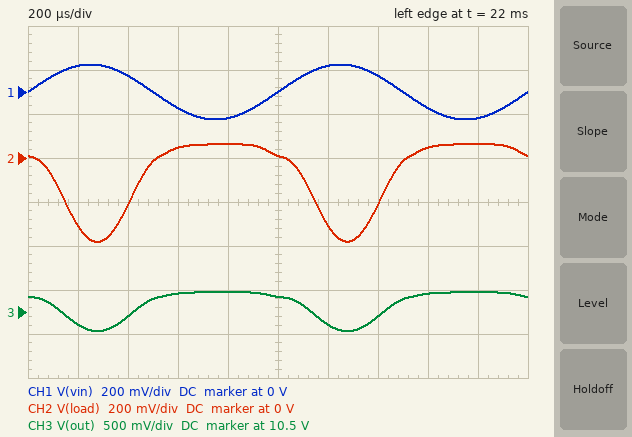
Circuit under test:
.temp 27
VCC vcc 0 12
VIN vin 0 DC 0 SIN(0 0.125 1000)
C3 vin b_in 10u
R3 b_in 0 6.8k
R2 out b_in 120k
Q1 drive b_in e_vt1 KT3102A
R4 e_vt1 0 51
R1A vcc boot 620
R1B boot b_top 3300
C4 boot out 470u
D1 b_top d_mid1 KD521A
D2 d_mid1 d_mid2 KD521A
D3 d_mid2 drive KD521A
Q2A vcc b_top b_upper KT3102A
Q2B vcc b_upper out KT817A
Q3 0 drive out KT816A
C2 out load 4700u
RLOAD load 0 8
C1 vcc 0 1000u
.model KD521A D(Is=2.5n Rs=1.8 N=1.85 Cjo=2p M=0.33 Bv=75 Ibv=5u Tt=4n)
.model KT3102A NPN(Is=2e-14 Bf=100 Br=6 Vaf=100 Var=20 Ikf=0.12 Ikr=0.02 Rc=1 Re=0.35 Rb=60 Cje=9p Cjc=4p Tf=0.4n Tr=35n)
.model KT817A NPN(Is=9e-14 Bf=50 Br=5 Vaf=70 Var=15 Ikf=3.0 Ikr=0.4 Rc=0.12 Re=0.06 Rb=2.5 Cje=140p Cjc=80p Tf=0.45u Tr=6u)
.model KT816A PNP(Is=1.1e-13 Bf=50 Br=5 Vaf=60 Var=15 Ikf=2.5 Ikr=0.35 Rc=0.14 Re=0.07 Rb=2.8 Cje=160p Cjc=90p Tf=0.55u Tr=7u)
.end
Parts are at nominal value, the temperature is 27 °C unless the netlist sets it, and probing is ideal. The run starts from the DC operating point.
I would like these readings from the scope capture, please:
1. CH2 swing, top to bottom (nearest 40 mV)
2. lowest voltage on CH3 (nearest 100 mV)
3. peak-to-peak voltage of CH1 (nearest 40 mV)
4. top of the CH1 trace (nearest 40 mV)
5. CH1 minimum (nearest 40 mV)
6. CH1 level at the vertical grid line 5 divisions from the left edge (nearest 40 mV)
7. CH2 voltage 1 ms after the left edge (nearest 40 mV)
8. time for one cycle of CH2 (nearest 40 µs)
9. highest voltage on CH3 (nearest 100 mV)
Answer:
440 mV
10.3 V
240 mV
120 mV
-120 mV
0 V
0 V
1.00 ms
10.7 V
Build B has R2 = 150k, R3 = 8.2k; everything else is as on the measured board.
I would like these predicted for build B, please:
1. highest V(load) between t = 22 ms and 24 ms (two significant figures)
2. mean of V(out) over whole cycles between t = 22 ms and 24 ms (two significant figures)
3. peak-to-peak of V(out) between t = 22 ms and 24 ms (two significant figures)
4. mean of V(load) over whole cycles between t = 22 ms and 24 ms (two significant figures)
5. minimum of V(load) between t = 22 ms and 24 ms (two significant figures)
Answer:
11 mV
11 V
340 mV
-78 mV
-330 mV
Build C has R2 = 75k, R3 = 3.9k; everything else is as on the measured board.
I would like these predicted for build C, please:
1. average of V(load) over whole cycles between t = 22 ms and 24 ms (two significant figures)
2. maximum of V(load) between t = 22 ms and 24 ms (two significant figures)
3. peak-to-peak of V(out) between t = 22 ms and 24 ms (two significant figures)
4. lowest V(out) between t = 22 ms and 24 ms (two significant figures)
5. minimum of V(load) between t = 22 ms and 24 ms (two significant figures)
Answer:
-53 mV
4.1 mV
240 mV
11 V
-240 mV
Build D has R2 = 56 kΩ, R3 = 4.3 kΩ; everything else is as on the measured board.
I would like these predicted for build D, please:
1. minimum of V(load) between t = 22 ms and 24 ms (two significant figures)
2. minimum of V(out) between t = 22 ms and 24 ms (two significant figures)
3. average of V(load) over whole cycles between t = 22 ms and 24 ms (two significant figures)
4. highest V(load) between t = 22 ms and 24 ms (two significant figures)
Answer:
-780 mV
8.7 V
430 mV
1.7 V
